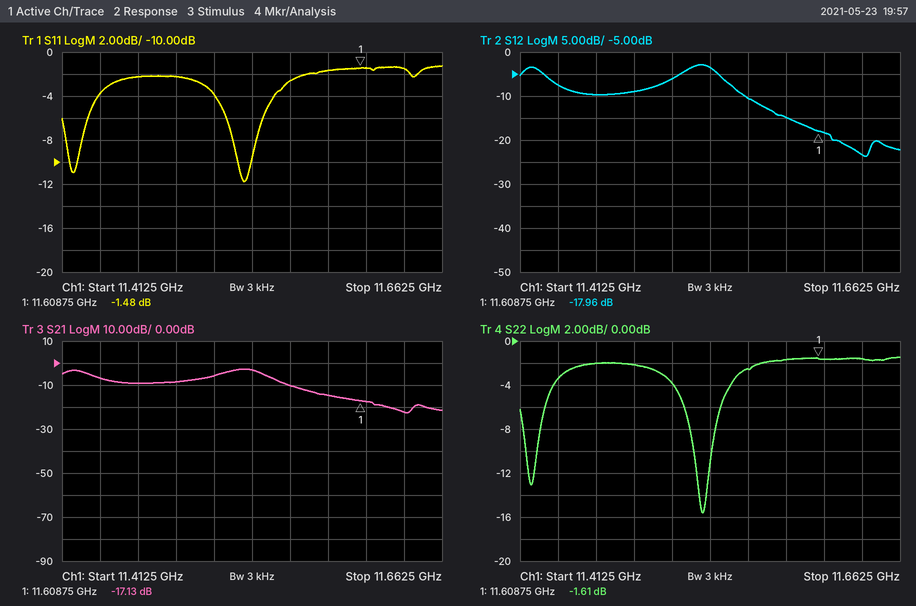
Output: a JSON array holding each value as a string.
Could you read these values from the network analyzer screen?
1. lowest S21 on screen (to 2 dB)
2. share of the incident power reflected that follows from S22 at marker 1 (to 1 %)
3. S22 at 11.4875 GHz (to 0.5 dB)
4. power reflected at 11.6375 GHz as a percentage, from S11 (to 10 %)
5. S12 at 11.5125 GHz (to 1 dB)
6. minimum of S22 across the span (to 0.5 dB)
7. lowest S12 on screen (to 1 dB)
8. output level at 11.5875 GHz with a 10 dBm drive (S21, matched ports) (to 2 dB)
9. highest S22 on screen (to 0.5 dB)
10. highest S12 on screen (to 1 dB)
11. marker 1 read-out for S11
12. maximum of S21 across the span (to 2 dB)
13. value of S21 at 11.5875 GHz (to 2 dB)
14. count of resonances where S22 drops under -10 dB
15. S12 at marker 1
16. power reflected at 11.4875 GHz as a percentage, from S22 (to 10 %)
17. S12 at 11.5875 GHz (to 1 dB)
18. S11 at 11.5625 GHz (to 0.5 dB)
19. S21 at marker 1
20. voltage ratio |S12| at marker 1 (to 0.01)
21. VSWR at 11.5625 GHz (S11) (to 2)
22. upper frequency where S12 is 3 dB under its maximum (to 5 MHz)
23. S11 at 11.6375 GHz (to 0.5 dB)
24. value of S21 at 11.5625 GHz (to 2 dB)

["-22 dB", "69 %", "-2.0 dB", "70 %", "-6 dB", "-15.5 dB", "-24 dB", "-4 dBm", "-1.5 dB", "-3 dB", "-1.48 dB", "-2 dB", "-14 dB", "2", "-17.96 dB", "60 %", "-15 dB", "-2.5 dB", "-17.13 dB", "0.13", "6", "11.545 GHz", "-1.5 dB", "-10 dB"]
